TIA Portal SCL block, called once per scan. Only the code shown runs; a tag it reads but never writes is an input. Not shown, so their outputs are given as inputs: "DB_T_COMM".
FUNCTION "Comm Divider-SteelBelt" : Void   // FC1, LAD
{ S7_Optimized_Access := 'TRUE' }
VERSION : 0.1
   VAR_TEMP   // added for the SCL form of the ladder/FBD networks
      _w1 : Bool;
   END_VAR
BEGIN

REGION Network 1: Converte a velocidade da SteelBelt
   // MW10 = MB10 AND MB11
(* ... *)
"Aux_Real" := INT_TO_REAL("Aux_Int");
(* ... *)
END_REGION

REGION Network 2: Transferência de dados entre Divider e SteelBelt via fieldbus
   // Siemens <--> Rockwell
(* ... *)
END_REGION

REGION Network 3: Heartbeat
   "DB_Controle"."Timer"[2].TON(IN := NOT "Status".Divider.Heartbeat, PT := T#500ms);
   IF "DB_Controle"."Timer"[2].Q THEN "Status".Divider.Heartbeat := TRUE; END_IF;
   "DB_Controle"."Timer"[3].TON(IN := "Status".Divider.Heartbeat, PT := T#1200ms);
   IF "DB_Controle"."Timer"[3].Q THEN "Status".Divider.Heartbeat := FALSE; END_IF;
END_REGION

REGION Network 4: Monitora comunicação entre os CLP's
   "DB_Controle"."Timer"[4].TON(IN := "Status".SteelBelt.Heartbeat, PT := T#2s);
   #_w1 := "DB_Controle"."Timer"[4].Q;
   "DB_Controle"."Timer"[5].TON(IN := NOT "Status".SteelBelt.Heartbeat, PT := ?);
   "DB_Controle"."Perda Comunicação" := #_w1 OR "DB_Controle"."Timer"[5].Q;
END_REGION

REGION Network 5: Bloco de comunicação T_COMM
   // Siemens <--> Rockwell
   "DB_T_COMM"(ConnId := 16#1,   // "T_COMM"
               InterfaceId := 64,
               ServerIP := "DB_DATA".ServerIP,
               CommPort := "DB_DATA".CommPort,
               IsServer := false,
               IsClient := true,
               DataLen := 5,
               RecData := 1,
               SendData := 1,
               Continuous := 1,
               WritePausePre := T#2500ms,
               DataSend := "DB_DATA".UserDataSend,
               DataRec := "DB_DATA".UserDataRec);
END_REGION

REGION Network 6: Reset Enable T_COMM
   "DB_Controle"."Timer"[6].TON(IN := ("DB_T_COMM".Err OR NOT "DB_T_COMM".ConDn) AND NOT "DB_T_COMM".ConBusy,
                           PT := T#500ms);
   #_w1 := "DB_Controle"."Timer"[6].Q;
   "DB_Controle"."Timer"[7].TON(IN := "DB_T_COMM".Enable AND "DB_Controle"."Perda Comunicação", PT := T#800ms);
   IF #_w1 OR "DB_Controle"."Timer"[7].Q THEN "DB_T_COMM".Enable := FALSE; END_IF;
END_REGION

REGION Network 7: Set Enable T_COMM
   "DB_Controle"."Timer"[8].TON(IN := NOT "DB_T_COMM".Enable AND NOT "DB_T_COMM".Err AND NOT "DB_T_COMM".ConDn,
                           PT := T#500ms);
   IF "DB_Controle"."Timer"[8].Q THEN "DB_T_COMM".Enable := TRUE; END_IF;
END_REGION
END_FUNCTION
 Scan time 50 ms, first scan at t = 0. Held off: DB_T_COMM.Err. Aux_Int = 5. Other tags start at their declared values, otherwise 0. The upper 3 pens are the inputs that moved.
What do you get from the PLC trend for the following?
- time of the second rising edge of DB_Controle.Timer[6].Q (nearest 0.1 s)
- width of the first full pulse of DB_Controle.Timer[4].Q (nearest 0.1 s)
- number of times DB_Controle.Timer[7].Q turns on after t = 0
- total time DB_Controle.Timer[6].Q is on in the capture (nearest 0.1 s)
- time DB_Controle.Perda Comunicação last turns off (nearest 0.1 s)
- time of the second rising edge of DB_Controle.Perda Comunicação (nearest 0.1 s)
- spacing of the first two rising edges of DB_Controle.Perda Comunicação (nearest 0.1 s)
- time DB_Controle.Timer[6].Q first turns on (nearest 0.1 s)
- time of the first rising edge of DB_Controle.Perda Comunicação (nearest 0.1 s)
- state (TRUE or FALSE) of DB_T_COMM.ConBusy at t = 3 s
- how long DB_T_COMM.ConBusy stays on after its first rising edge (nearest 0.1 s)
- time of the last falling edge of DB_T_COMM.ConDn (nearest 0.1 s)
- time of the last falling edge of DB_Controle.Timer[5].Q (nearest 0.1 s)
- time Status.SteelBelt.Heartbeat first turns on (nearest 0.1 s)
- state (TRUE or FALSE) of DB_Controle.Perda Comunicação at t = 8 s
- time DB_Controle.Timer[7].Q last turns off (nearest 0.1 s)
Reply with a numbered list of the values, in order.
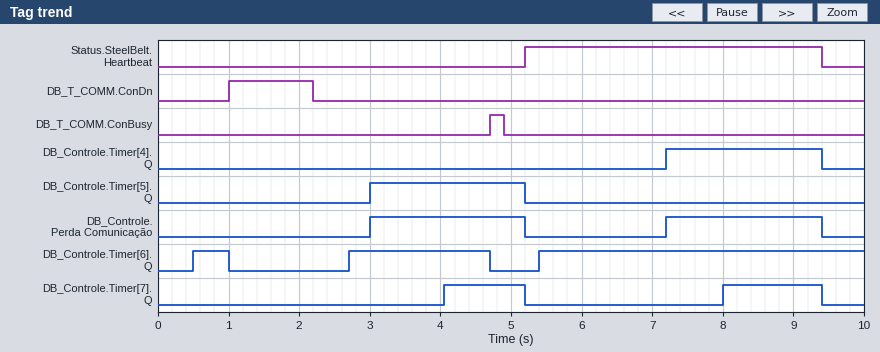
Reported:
1. 2.7 s
2. 2.2 s
3. 2
4. 7.1 s
5. 9.4 s
6. 7.2 s
7. 4.2 s
8. 0.5 s
9. 3.0 s
10. FALSE
11. 0.2 s
12. 2.2 s
13. 5.2 s
14. 5.2 s
15. TRUE
16. 9.4 s
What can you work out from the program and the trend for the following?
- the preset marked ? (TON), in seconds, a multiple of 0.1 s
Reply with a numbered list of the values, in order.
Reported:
1. 3.0 s
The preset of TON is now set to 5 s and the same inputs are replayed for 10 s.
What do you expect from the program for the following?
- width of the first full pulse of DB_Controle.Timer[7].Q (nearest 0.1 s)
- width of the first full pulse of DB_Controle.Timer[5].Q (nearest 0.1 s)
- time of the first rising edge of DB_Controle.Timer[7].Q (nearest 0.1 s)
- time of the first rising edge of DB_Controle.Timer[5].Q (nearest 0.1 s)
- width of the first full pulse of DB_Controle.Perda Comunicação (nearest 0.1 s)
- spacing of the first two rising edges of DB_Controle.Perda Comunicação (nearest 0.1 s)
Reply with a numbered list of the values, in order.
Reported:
1. 1.4 s
2. 0.2 s
3. 8.0 s
4. 5.0 s
5. 0.2 s
6. 2.2 s
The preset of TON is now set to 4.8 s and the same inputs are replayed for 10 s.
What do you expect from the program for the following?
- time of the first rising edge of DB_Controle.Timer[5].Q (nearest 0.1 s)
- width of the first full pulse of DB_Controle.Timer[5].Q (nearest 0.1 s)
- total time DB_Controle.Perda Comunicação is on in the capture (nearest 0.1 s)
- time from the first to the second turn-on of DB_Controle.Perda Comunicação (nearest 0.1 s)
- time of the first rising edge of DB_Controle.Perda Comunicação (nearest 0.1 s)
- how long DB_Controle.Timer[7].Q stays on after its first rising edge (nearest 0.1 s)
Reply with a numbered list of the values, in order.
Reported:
1. 4.8 s
2. 0.4 s
3. 2.6 s
4. 2.4 s
5. 4.8 s
6. 1.4 s
